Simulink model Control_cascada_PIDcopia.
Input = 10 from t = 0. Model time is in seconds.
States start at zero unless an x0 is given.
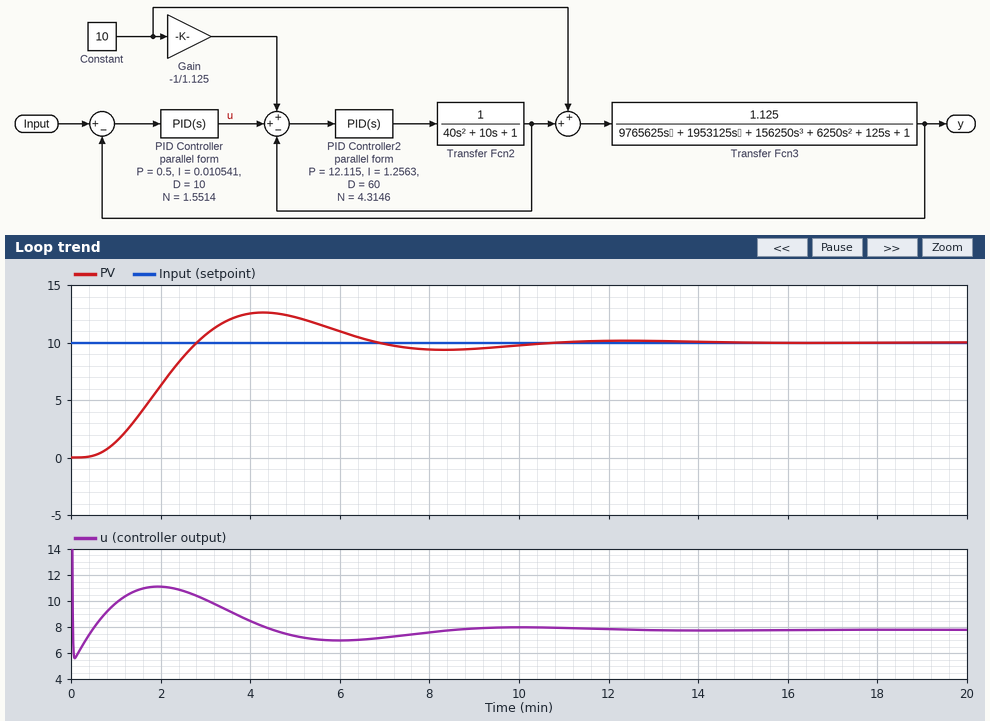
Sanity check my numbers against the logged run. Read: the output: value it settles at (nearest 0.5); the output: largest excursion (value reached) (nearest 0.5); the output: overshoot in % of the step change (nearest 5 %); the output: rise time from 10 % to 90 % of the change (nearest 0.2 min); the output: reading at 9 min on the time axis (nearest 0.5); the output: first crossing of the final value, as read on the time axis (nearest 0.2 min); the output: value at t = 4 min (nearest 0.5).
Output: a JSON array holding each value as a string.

["10.0", "12.5", "25 %", "1.6 min", "9.5", "2.8 min", "12.5"]
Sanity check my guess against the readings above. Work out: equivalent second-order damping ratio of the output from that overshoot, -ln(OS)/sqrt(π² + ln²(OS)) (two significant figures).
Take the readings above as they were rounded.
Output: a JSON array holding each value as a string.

["0.40"]
